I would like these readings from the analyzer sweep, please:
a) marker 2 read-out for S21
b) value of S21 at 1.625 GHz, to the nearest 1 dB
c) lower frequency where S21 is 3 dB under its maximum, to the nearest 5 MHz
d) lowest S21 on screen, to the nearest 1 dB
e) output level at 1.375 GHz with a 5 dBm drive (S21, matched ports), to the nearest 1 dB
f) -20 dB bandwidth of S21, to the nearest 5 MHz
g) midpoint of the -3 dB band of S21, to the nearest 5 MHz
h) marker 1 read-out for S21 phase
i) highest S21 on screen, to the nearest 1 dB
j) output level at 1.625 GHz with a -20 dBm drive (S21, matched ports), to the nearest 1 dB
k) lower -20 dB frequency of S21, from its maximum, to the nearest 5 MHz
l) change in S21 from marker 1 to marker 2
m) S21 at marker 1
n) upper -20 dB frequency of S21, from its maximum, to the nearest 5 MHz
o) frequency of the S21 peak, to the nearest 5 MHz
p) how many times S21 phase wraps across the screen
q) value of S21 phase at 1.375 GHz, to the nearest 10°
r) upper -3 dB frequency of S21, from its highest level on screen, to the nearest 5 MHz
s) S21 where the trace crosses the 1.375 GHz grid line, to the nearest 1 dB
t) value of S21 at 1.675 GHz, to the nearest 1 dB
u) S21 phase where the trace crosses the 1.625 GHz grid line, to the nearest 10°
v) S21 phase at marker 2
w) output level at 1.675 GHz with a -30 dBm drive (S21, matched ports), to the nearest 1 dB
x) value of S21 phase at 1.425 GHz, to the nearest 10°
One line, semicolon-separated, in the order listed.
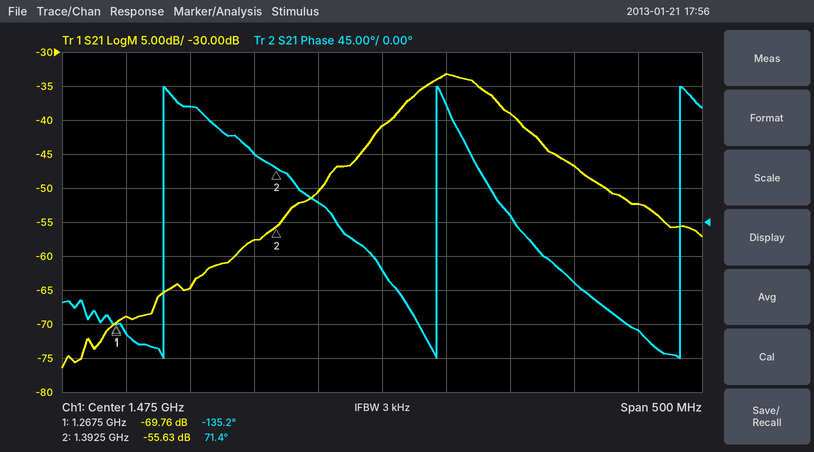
-55.63 dB; -47 dB; 1.500 GHz; -76 dB; -53 dBm; 280 MHz; 1.530 GHz; -135.2°; -33 dB; -67 dBm; 1.405 GHz; 14.13 dB; -69.76 dB; 1.685 GHz; 1.525 GHz; 3; 90°; 1.560 GHz; -58 dB; -52 dB; -80°; 71.4°; -82 dBm; 30°
